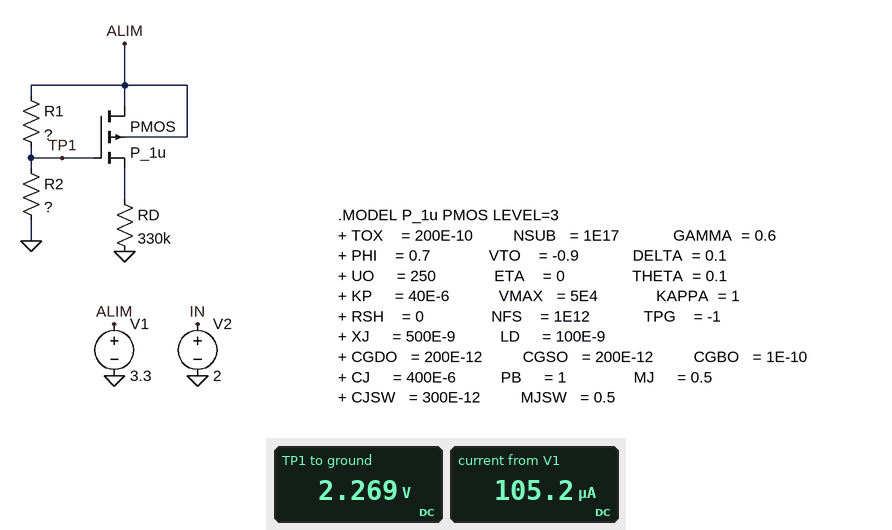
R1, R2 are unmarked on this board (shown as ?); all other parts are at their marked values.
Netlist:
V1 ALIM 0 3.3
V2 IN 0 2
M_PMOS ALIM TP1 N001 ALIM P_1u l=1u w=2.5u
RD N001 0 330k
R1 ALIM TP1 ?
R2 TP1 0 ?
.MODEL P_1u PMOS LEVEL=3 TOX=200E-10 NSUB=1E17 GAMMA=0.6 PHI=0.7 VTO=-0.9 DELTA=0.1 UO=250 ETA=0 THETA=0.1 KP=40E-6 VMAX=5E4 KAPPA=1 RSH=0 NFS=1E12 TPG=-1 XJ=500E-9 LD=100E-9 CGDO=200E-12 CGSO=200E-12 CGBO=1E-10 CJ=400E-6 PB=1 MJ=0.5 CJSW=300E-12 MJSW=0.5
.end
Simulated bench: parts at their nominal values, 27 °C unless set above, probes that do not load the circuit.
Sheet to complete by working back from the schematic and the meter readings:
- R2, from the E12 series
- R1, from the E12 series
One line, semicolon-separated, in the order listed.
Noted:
22 kΩ; 10 kΩ
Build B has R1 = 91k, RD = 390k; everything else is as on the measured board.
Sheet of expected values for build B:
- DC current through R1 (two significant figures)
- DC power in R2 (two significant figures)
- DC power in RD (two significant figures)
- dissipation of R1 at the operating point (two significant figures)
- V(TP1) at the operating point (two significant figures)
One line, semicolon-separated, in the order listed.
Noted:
29 µA; 19 µW; 27 µW; 78 µW; 640 mV
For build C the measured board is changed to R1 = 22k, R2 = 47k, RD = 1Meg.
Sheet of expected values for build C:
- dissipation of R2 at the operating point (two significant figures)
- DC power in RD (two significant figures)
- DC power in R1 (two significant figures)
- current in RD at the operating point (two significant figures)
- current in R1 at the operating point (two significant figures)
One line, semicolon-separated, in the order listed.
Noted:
110 µW; 5.3 µW; 50 µW; 2.3 µA; 48 µA
